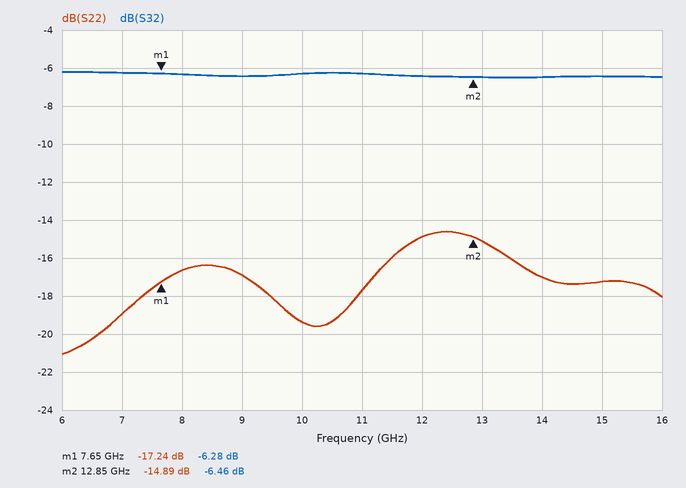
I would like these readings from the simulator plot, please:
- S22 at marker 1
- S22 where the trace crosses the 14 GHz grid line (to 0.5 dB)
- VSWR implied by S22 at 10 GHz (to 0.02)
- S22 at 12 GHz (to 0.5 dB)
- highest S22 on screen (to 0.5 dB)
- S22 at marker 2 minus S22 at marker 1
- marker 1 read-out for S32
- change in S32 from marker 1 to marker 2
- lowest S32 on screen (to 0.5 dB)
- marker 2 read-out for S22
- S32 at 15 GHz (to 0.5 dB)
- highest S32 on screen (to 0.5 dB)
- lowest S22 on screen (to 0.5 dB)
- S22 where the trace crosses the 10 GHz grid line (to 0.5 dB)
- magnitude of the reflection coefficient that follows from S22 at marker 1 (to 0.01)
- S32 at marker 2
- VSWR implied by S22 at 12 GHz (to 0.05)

-17.24 dB
-17.0 dB
1.24
-15.0 dB
-14.5 dB
2.35 dB
-6.28 dB
-0.18 dB
-6.5 dB
-14.89 dB
-6.5 dB
-6.0 dB
-21.0 dB
-19.5 dB
0.14
-6.46 dB
1.45
